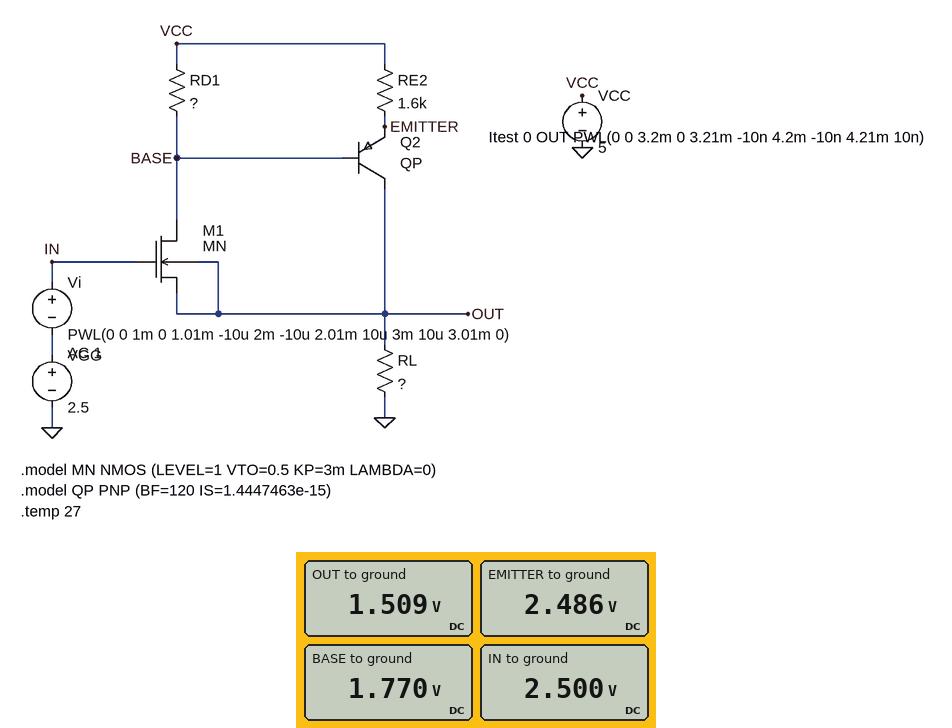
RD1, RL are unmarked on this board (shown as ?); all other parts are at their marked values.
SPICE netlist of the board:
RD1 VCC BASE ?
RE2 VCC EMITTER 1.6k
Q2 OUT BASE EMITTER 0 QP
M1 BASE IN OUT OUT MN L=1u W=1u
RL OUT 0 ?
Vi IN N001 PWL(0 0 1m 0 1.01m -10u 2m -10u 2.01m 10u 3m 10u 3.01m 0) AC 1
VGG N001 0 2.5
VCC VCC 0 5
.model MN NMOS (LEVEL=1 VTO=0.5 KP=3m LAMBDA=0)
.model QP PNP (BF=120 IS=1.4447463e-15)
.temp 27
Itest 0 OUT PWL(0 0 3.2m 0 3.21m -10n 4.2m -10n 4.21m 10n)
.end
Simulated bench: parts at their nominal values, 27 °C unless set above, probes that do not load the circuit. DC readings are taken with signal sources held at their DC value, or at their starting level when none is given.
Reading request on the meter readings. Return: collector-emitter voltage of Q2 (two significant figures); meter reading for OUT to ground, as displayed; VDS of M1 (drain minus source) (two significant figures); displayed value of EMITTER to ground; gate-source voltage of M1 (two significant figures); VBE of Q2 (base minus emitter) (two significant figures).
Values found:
-980 mV
1.509 V
260 mV
2.486 V
990 mV
-720 mV
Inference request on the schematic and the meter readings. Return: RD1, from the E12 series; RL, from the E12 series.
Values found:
12 kΩ
820 Ω
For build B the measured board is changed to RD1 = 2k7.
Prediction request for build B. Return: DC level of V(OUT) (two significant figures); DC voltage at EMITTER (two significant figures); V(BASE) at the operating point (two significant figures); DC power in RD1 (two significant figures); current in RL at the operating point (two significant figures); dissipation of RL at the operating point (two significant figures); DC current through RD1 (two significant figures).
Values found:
1.3 V
3.7 V
3.0 V
1.5 mW
1.6 mA
2.0 mW
750 µA
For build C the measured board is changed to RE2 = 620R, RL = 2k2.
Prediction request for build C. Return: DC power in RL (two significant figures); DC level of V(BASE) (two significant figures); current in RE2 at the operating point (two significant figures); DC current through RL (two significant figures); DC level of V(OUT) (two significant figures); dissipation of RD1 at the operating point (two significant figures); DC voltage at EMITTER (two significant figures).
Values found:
1.4 mW
3.9 V
700 µA
790 µA
1.7 V
110 µW
4.6 V
